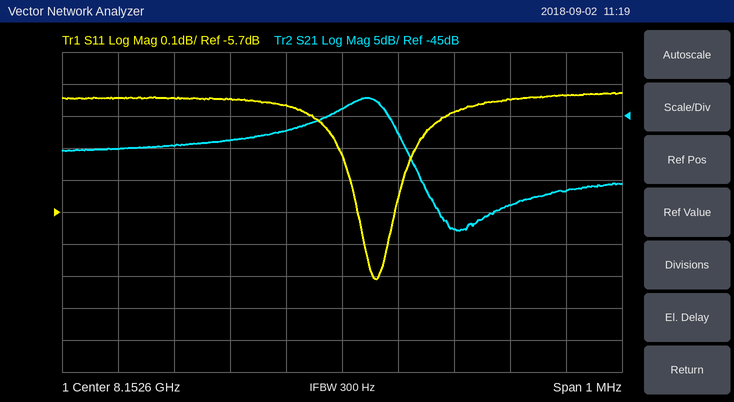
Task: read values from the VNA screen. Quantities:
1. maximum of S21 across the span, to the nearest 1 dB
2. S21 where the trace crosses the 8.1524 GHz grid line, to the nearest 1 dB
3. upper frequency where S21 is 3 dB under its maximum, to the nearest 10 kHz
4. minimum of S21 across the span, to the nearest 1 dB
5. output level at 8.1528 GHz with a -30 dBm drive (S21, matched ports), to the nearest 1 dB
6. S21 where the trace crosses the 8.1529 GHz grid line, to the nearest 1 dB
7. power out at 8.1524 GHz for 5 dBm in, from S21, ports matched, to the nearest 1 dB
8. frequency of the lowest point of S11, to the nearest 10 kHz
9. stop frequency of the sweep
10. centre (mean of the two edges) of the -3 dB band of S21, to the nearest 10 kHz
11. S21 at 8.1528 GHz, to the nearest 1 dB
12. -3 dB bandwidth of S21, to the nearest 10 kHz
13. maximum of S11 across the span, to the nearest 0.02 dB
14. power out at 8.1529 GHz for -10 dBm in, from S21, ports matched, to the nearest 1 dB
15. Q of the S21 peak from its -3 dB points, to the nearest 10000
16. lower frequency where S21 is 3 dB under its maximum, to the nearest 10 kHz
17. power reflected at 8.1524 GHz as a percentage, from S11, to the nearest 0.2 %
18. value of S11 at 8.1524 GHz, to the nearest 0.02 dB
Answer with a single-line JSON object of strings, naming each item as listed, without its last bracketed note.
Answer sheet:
{"maximum of S21 across the span, to the nearest 1 dB": "-42 dB", "S21 where the trace crosses the 8.1524 GHz grid line, to the nearest 1 dB": "-49 dB", "upper frequency where S21 is 3 dB under its maximum, to the nearest 10 kHz": "8.15268 GHz", "minimum of S21 across the span, to the nearest 1 dB": "-63 dB", "output level at 8.1528 GHz with a -30 dBm drive (S21, matched ports), to the nearest 1 dB": "-93 dBm", "S21 where the trace crosses the 8.1529 GHz grid line, to the nearest 1 dB": "-59 dB", "power out at 8.1524 GHz for 5 dBm in, from S21, ports matched, to the nearest 1 dB": "-44 dBm", "frequency of the lowest point of S11, to the nearest 10 kHz": "8.15266 GHz", "stop frequency of the sweep": "8.1531 GHz", "centre (mean of the two edges) of the -3 dB band of S21, to the nearest 10 kHz": "8.15263 GHz", "S21 at 8.1528 GHz, to the nearest 1 dB": "-63 dB", "-3 dB bandwidth of S21, to the nearest 10 kHz": "110 kHz", "maximum of S11 across the span, to the nearest 0.02 dB": "-5.32 dB", "power out at 8.1529 GHz for -10 dBm in, from S21, ports matched, to the nearest 1 dB": "-69 dBm", "Q of the S21 peak from its -3 dB points, to the nearest 10000": "70000", "lower frequency where S21 is 3 dB under its maximum, to the nearest 10 kHz": "8.15257 GHz", "power reflected at 8.1524 GHz as a percentage, from S11, to the nearest 0.2 %": "29.2 %", "value of S11 at 8.1524 GHz, to the nearest 0.02 dB": "-5.34 dB"}
